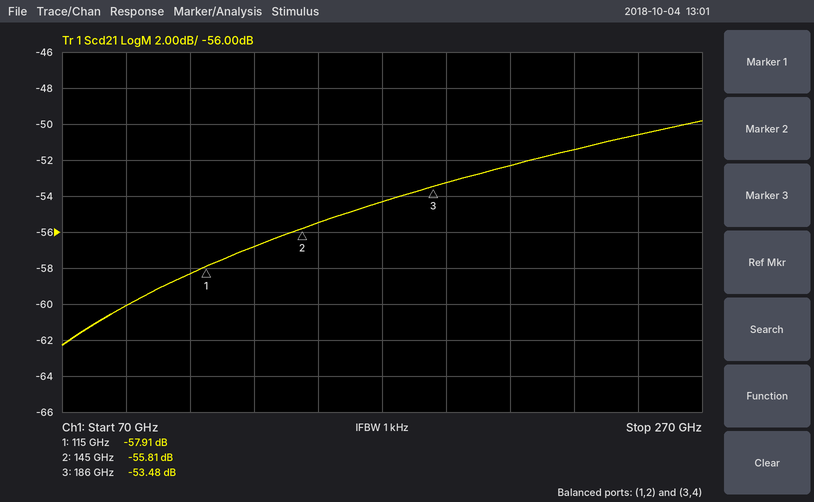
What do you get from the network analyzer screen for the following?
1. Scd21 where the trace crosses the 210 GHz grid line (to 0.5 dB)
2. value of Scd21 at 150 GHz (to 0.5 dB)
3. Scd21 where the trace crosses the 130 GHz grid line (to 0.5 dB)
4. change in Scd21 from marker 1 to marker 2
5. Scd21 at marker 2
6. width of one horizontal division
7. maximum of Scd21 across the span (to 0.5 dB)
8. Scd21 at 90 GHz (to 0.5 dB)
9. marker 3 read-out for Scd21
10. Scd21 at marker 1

-52.5 dB
-55.5 dB
-57.0 dB
2.10 dB
-55.81 dB
20 GHz
-50.0 dB
-60.0 dB
-53.48 dB
-57.91 dB
